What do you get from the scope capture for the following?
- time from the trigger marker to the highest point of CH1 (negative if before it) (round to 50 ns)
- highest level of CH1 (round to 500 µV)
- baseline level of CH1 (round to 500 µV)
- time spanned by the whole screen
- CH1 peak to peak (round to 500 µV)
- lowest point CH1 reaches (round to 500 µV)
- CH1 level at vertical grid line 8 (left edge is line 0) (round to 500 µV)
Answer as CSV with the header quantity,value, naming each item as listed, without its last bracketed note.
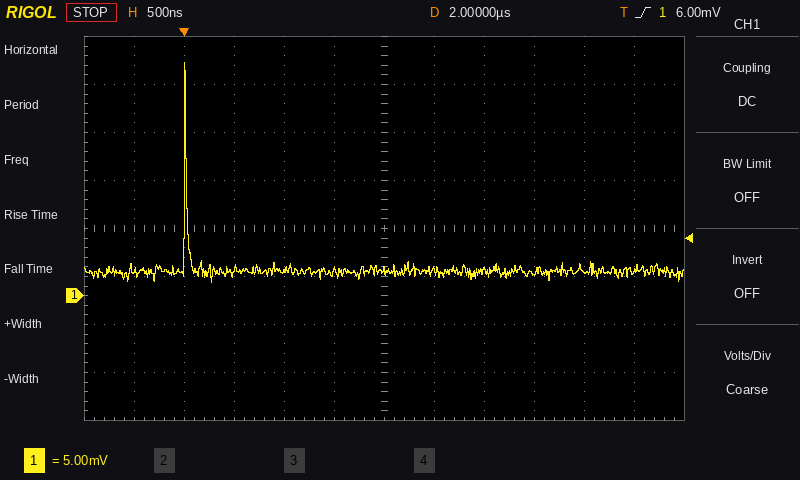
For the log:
quantity,value
time from the trigger marker to the highest point of CH1 (negative if before it),0 ns
highest level of CH1,24.5 mV
baseline level of CH1,2.5 mV
time spanned by the whole screen,6 µs
CH1 peak to peak,23.0 mV
lowest point CH1 reaches,1.5 mV
CH1 level at vertical grid line 8 (left edge is line 0),2.5 mV
